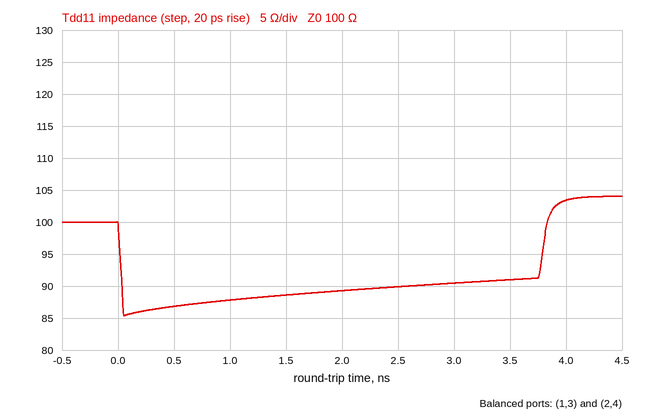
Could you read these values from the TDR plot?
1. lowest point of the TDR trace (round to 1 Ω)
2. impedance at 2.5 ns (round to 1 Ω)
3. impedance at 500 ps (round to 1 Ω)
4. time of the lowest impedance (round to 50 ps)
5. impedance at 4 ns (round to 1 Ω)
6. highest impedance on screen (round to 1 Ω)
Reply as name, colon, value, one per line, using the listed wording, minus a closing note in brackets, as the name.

lowest point of the TDR trace: 85 Ω
impedance at 2.5 ns: 90 Ω
impedance at 500 ps: 87 Ω
time of the lowest impedance: 50 ps
impedance at 4 ns: 103 Ω
highest impedance on screen: 104 Ω
